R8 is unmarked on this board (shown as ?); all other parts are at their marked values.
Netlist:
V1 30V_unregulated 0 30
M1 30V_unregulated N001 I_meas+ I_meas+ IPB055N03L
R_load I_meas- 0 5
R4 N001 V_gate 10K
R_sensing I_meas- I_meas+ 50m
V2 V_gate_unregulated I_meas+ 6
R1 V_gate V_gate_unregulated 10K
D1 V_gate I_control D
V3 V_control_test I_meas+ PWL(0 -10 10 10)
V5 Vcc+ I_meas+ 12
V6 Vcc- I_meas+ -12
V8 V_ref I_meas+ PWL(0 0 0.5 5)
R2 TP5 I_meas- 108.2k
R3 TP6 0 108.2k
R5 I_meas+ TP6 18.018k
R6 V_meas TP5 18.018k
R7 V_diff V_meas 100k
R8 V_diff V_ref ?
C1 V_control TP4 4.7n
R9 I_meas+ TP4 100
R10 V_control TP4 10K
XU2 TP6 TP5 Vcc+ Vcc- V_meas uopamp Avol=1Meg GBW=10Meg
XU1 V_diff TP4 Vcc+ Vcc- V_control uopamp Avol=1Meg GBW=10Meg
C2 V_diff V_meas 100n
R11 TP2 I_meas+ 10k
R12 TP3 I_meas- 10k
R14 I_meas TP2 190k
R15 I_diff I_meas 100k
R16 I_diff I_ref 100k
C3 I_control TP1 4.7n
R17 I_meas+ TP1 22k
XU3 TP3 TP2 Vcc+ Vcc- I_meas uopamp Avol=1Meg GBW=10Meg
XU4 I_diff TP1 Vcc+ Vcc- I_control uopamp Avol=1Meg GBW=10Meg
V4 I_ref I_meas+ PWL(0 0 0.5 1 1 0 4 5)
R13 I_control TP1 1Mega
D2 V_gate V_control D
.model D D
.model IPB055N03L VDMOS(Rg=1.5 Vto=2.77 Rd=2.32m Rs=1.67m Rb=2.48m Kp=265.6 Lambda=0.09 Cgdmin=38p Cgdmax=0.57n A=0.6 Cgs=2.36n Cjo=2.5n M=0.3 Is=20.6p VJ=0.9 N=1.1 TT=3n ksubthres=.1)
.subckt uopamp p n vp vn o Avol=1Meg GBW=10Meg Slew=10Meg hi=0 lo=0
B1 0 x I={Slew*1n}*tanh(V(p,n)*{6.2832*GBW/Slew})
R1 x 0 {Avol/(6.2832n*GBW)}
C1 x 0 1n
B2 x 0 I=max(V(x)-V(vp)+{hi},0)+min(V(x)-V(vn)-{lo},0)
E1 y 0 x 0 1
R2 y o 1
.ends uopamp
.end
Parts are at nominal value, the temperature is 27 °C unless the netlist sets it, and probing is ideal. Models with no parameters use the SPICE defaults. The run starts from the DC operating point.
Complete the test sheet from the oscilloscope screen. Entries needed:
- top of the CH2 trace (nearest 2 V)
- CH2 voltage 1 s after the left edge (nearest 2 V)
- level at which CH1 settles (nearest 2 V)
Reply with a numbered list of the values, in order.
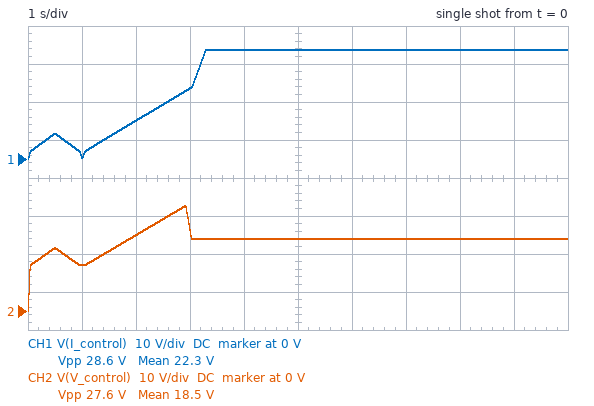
1. 28 V
2. 12 V
3. 28 V
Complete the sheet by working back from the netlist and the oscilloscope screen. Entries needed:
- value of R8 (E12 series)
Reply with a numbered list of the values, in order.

1. 180 kΩ
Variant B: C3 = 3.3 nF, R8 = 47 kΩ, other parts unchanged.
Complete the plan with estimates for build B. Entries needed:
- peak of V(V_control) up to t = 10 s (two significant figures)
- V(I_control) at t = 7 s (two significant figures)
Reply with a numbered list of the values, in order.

1. 37 V
2. 27 V
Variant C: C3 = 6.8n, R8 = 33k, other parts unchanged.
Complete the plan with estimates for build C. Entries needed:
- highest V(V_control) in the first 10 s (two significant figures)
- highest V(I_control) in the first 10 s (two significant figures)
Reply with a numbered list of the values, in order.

1. 37 V
2. 27 V
